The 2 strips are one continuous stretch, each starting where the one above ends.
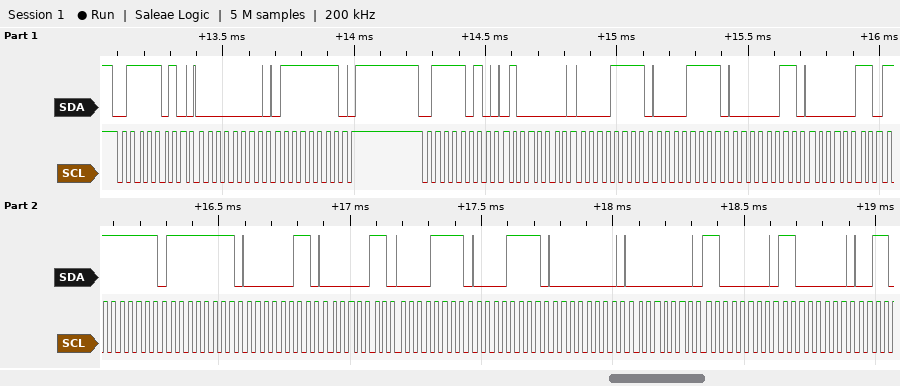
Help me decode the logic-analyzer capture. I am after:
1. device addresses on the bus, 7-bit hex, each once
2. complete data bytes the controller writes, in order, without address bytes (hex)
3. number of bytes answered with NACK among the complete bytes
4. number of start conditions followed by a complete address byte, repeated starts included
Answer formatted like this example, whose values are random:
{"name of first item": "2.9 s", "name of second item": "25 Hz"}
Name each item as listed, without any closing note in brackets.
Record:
{"device addresses on the bus, 7-bit hex, each once": "0x3D", "complete data bytes the controller writes, in order, without address bytes": "00 7F 40 0F 0F 03 03 FF FF 03 03 0F 0F 00 00 C0 C0", "number of bytes answered with NACK among the complete bytes": "0", "number of start conditions followed by a complete address byte, repeated starts included": "2"}
